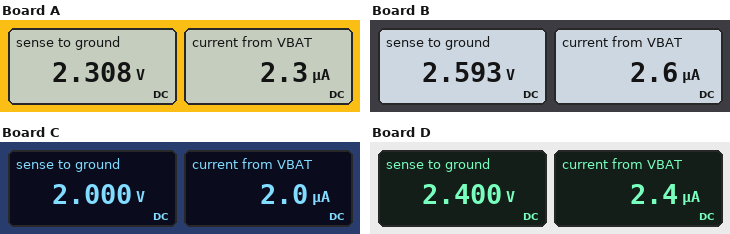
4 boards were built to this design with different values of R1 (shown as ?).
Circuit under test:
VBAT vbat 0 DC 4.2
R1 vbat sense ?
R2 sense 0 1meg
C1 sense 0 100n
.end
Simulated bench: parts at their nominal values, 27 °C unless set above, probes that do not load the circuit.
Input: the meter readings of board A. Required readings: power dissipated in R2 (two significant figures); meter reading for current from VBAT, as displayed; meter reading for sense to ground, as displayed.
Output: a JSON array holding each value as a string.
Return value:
["5.3 µW", "2.3 µA", "2.308 V"]
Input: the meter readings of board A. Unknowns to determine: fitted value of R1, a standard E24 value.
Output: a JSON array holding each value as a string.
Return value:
["820 kΩ"]
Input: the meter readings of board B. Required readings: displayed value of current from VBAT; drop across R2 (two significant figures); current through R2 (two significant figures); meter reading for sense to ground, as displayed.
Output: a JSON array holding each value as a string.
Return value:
["2.6 µA", "2.6 V", "2.6 µA", "2.593 V"]
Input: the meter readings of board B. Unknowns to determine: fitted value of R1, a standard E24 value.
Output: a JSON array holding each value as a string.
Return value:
["620 kΩ"]
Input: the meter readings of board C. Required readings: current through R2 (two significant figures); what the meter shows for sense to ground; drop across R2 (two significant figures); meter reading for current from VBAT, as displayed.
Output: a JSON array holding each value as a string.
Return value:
["2.0 µA", "2.000 V", "2.0 V", "2.0 µA"]
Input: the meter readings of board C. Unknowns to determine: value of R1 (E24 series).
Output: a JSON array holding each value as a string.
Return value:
["1.1 MΩ"]
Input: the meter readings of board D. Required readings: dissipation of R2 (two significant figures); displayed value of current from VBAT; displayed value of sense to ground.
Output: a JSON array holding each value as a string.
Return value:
["5.8 µW", "2.4 µA", "2.400 V"]
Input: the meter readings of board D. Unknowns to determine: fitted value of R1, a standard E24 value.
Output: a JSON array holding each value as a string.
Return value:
["750 kΩ"]
